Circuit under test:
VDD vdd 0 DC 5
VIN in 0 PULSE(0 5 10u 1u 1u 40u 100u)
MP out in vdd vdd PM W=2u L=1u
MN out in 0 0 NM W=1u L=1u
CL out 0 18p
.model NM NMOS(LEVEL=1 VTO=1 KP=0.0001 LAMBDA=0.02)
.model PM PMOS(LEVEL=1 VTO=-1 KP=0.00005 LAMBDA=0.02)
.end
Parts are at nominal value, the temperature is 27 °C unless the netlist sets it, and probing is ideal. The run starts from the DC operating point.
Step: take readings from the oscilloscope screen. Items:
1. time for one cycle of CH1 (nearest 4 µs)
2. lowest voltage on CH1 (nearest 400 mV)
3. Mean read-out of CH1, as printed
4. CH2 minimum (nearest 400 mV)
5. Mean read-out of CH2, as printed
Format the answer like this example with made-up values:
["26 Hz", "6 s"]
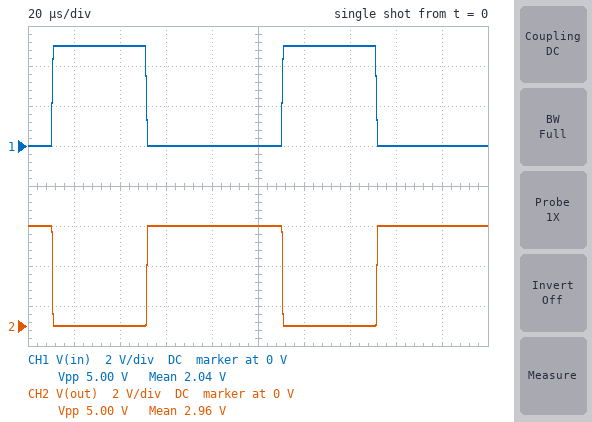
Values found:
["100 µs", "0 V", "2.04 V", "0 V", "2.96 V"]
